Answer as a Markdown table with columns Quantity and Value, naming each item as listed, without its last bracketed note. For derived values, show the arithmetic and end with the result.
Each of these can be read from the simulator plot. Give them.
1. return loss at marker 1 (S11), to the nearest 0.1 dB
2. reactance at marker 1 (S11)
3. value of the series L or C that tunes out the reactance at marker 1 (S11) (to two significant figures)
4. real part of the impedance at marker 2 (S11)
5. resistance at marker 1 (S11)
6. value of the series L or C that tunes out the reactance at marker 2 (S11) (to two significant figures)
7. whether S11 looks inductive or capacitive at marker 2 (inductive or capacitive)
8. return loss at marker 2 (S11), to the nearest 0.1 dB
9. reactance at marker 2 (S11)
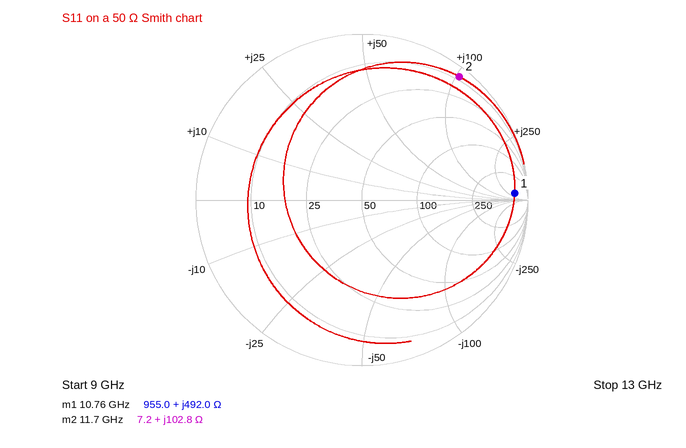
| Quantity | Value |
|---|---|
| return loss at marker 1 (S11), to the nearest 0.1 dB | 0.7 dB |
| reactance at marker 1 | +492.0 Ω |
| value of the series L or C that tunes out the reactance at marker 1 (S11) | C = 1/(2π × 10.76 GHz × 492 Ω) ≈ 30 fF |
| real part of the impedance at marker 2 | 7.2 Ω |
| resistance at marker 1 | 955.0 Ω |
| value of the series L or C that tunes out the reactance at marker 2 (S11) | C = 1/(2π × 11.7 GHz × 102.8 Ω) ≈ 132 fF, so 130 fF to two significant figures |
| whether S11 looks inductive or capacitive at marker 2 | inductive |
| return loss at marker 2 (S11), to the nearest 0.1 dB | 0.5 dB |
| reactance at marker 2 | +102.8 Ω |
